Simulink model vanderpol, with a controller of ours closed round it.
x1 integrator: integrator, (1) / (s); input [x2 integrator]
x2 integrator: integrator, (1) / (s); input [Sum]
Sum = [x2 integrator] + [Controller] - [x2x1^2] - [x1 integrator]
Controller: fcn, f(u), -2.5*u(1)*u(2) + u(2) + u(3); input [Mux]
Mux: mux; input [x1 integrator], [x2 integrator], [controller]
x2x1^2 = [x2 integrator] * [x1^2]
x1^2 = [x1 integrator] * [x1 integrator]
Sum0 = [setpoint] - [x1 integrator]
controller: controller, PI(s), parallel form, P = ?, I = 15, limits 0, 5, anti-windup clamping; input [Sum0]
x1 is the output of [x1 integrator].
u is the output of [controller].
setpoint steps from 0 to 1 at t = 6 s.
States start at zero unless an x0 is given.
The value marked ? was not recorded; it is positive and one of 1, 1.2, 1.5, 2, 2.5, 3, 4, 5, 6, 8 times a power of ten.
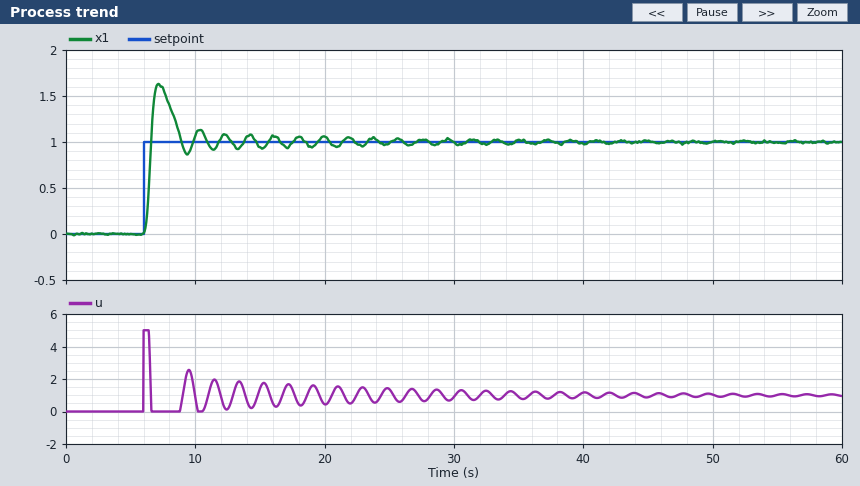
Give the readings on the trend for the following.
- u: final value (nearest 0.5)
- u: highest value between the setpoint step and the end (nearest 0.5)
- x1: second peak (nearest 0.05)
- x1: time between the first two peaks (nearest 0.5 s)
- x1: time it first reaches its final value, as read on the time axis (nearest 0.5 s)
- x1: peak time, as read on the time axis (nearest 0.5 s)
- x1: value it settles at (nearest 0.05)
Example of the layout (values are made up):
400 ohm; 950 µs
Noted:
1.0; 5.0; 1.15; 3.0 s; 6.5 s; 7.0 s; 1.00
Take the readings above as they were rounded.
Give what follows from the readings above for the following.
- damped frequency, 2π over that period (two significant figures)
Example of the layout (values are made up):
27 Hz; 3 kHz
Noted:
2.1 rad/s
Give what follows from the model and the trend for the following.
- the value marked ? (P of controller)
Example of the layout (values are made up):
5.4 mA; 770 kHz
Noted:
10
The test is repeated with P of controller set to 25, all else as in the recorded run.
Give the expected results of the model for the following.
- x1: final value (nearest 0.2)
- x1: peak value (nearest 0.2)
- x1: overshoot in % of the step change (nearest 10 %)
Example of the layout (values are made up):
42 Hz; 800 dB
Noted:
1.0; 1.6; 70 %
